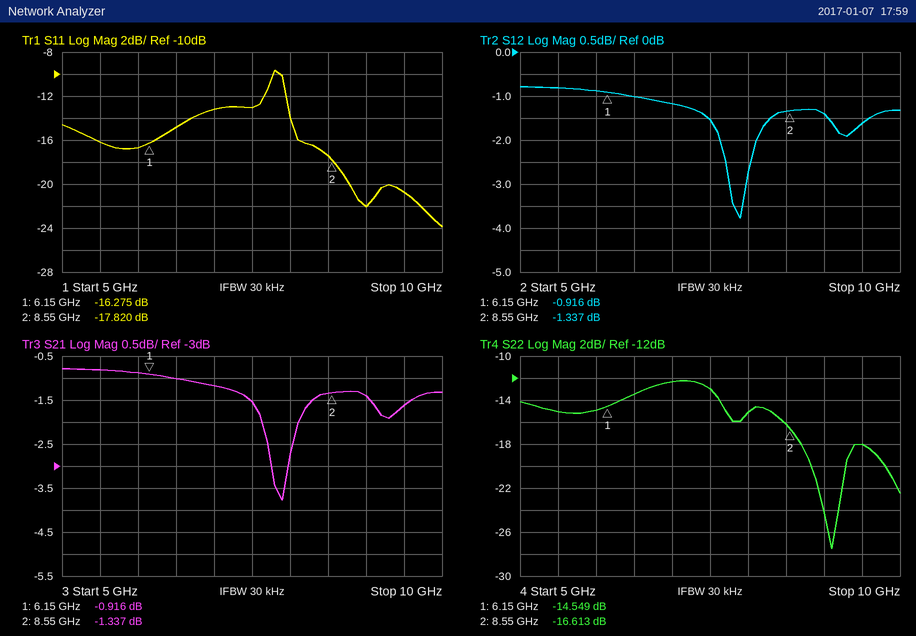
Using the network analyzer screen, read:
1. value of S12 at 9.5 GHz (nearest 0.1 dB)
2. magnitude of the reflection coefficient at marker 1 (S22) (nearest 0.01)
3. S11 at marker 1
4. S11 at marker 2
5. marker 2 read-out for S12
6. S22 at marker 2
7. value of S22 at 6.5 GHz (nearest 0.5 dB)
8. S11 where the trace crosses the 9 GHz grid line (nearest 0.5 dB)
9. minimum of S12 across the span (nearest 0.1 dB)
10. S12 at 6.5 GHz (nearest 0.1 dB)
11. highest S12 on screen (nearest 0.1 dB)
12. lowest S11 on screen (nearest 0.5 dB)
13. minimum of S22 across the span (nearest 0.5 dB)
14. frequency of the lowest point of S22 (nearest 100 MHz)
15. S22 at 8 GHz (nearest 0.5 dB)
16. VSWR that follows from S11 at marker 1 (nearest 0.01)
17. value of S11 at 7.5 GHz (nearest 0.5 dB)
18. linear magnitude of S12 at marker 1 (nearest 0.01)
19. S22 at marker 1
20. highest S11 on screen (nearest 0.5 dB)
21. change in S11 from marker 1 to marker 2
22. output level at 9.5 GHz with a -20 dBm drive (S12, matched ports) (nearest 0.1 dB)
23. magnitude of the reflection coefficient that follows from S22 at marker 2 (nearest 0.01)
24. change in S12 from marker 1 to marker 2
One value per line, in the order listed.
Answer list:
-1.6 dB
0.19
-16.275 dB
-17.820 dB
-1.337 dB
-16.613 dB
-13.5 dB
-22.0 dB
-3.8 dB
-1.0 dB
-0.8 dB
-24.0 dB
-27.5 dB
9.1 GHz
-15.0 dB
1.36
-13.0 dB
0.90
-14.549 dB
-9.5 dB
-1.545 dB
-21.6 dBm
0.15
-0.421 dB
